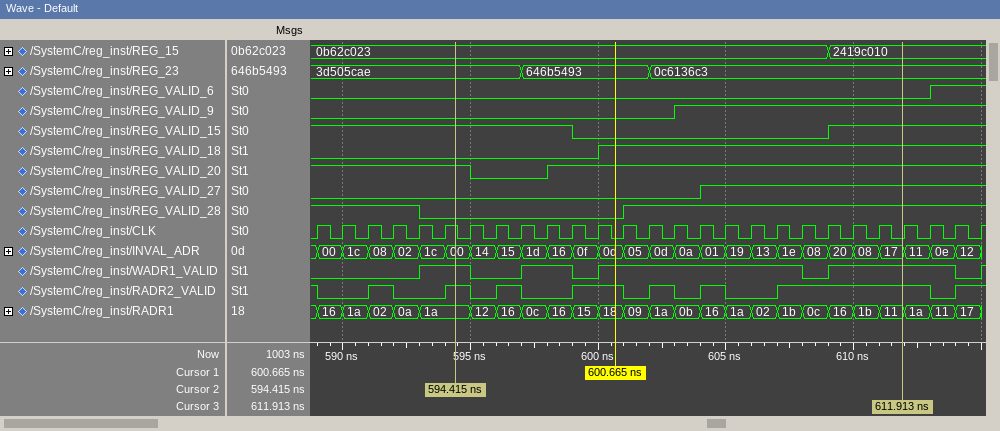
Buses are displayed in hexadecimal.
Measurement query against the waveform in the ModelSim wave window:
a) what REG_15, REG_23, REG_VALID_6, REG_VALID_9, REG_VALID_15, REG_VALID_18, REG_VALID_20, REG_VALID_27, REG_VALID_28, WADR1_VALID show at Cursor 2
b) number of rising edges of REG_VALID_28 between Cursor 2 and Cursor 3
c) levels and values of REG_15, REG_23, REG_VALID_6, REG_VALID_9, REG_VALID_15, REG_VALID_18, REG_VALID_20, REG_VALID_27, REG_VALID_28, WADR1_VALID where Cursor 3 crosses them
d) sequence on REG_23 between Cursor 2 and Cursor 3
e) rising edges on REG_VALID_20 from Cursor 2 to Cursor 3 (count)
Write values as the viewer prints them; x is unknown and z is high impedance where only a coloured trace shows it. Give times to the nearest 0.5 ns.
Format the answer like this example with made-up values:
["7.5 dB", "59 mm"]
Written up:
["REG_15=0b62c023, REG_23=3d505cae, REG_VALID_6=0, REG_VALID_9=0, REG_VALID_15=1, REG_VALID_18=0, REG_VALID_20=1, REG_VALID_27=0, REG_VALID_28=0, WADR1_VALID=1", "1", "REG_15=2419c010, REG_23=0c6136c3, REG_VALID_6=0, REG_VALID_9=1, REG_VALID_15=1, REG_VALID_18=1, REG_VALID_20=1, REG_VALID_27=1, REG_VALID_28=1, WADR1_VALID=1", "3d505cae, 646b5493, 0c6136c3", "1"]
